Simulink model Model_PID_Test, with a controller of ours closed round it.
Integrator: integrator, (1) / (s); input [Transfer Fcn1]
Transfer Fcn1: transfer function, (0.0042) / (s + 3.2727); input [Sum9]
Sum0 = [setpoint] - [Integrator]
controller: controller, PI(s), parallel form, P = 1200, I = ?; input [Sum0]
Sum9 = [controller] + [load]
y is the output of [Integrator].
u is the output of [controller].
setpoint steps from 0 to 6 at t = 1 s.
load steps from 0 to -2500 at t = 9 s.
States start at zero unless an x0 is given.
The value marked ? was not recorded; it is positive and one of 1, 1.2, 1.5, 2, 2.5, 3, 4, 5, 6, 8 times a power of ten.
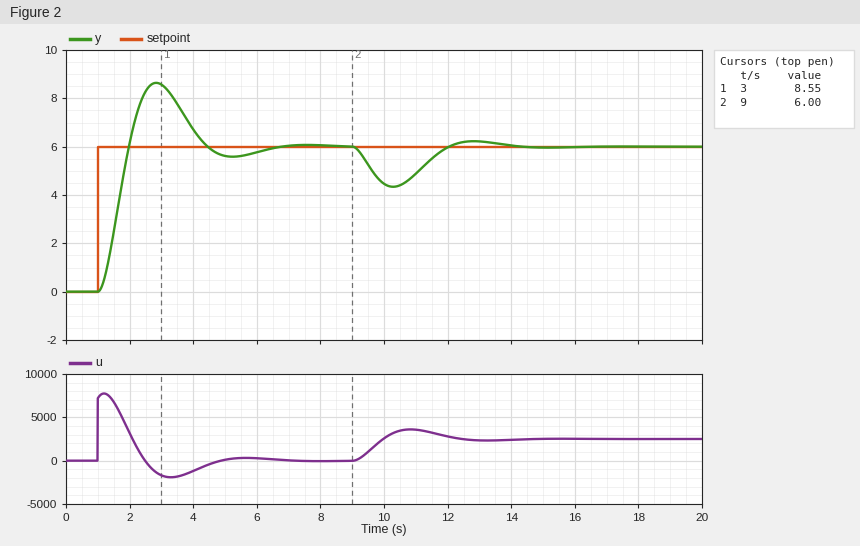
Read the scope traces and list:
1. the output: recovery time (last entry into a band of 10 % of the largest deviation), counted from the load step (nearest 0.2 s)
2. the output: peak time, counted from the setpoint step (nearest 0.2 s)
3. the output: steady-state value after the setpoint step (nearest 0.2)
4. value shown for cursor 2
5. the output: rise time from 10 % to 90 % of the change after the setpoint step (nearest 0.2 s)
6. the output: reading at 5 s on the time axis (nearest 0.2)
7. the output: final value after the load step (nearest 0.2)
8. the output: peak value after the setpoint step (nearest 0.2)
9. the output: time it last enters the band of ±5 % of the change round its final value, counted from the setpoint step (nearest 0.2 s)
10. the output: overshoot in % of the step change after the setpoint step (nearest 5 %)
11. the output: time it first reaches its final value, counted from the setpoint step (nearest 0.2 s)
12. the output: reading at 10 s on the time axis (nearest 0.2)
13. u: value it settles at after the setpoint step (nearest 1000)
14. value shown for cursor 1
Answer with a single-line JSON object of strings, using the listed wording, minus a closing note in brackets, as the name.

{"the output: recovery time (last entry into a band of 10 % of the largest deviation), counted from the load step": "4.4 s", "the output: peak time, counted from the setpoint step": "1.8 s", "the output: steady-state value after the setpoint step": "6.0", "value shown for cursor 2": "6.00", "the output: rise time from 10 % to 90 % of the change after the setpoint step": "0.6 s", "the output: reading at 5 s on the time axis": "5.6", "the output: final value after the load step": "6.0", "the output: peak value after the setpoint step": "8.6", "the output: time it last enters the band of ±5 % of the change round its final value, counted from the setpoint step": "4.8 s", "the output: overshoot in % of the step change after the setpoint step": "45 %", "the output: time it first reaches its final value, counted from the setpoint step": "1.0 s", "the output: reading at 10 s on the time axis": "4.4", "u: value it settles at after the setpoint step": "0", "value shown for cursor 1": "8.55"}
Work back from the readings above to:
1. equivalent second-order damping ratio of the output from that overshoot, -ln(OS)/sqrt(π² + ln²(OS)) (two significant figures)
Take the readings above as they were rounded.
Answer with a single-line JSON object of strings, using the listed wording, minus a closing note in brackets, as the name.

{"equivalent second-order damping ratio of the output from that overshoot, -ln(OS)/sqrt(π² + ln²(OS))": "0.25"}
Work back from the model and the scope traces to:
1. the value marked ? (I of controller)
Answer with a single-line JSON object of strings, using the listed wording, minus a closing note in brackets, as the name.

{"the value marked ?": "1000"}
